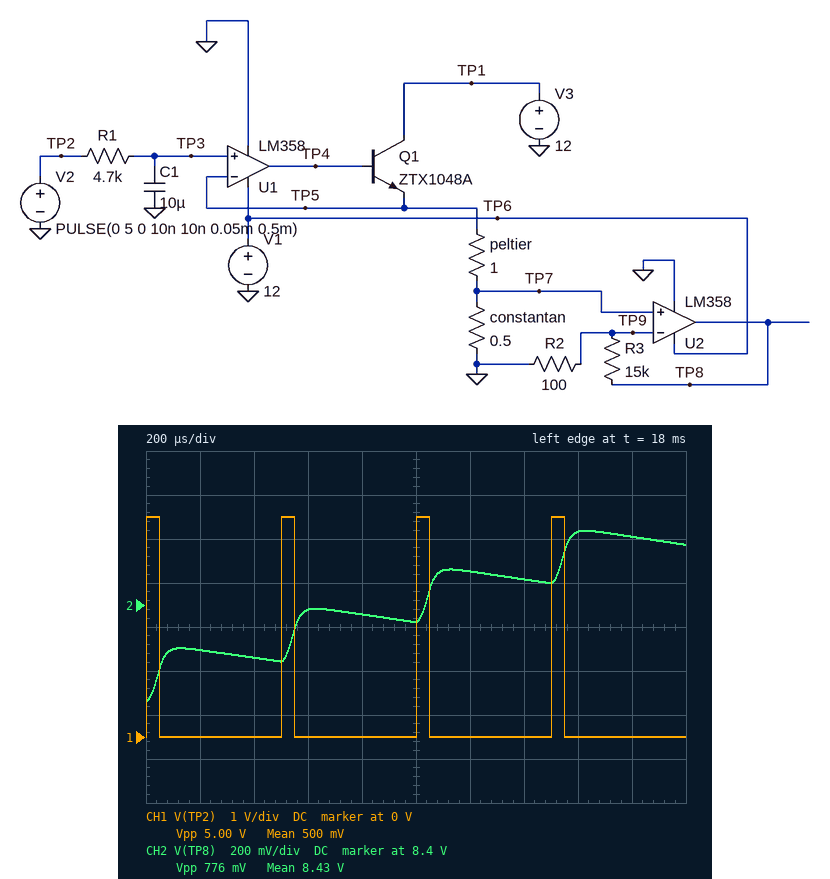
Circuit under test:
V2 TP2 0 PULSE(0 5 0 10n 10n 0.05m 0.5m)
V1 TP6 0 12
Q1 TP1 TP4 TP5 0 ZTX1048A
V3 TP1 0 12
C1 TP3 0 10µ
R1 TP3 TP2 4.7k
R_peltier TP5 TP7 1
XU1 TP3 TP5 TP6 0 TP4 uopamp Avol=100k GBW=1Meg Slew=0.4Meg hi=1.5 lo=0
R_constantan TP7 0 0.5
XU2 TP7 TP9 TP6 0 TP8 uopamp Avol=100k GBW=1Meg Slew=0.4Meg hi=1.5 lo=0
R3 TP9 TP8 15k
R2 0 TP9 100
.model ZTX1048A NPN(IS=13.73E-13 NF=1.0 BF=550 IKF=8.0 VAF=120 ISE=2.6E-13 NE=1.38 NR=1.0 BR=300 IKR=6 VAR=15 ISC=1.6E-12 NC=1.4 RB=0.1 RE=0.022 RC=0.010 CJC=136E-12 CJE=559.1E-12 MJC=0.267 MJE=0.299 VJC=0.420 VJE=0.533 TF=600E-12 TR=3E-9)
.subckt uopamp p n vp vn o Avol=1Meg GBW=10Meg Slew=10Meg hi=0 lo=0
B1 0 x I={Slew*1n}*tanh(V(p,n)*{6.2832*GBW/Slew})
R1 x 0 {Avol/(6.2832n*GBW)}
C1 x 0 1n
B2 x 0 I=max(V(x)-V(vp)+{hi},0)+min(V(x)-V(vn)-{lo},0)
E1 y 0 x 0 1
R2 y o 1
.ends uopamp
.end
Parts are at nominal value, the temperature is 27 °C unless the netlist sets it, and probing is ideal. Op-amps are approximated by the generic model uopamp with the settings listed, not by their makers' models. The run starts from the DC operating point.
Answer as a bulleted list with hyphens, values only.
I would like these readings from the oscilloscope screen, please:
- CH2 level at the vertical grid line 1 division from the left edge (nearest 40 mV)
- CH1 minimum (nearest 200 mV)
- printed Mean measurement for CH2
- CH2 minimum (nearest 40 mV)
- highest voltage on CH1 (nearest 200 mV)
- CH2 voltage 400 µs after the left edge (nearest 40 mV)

- 8.20 V
- 0 V
- 8.43 V
- 7.96 V
- 5.0 V
- 8.16 V
